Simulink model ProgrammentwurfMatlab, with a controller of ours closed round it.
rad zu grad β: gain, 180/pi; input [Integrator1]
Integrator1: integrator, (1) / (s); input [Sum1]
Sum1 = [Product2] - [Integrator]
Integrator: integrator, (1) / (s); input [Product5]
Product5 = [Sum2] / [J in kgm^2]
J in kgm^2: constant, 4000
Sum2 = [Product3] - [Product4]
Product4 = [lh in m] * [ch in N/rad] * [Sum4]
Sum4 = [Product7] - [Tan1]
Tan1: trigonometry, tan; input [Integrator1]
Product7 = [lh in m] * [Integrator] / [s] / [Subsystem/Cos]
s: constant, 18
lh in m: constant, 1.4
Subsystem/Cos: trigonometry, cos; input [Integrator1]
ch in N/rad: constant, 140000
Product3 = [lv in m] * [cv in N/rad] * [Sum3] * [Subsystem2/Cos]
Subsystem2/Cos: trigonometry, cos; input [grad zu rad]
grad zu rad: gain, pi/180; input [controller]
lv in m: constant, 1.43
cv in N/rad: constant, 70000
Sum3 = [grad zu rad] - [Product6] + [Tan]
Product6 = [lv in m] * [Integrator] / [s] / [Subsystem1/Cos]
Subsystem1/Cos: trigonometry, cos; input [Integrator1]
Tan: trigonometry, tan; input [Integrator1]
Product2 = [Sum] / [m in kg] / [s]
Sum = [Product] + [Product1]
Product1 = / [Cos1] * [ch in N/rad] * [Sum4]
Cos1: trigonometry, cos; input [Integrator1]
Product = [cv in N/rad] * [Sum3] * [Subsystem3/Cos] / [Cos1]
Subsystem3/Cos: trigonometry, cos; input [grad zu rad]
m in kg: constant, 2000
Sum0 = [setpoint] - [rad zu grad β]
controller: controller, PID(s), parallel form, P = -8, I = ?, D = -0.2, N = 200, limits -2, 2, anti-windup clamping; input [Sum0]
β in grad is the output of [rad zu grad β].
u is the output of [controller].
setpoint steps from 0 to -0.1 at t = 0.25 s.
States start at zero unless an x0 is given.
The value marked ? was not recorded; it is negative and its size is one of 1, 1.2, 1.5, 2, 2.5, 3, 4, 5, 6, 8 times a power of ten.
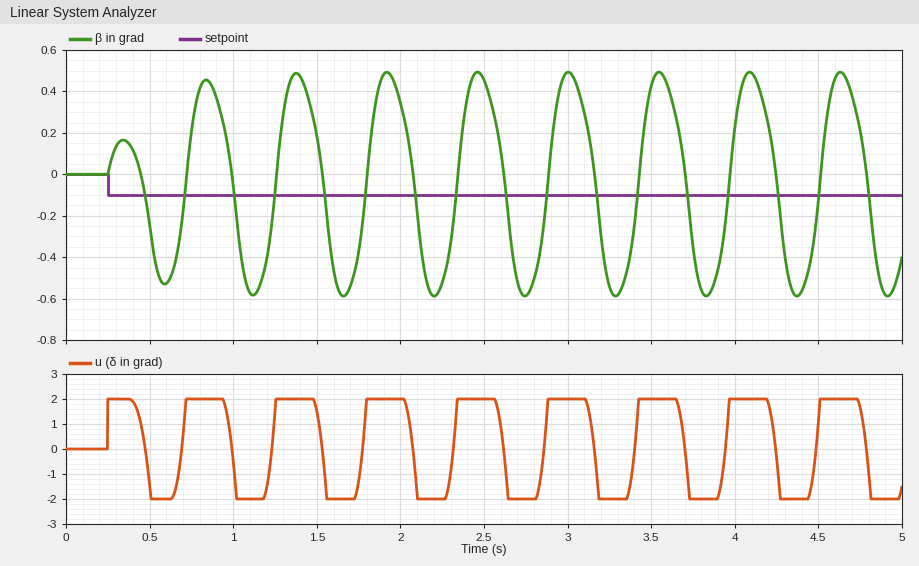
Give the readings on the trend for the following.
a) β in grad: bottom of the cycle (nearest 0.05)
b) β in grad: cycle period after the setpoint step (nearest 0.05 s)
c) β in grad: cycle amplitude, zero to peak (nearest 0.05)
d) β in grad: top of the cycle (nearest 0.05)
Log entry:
-0.60
0.55 s
0.55
0.50
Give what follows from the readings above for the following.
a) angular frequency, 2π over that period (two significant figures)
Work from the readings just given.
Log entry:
11 rad/s
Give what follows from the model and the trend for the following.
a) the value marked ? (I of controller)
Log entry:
-50
